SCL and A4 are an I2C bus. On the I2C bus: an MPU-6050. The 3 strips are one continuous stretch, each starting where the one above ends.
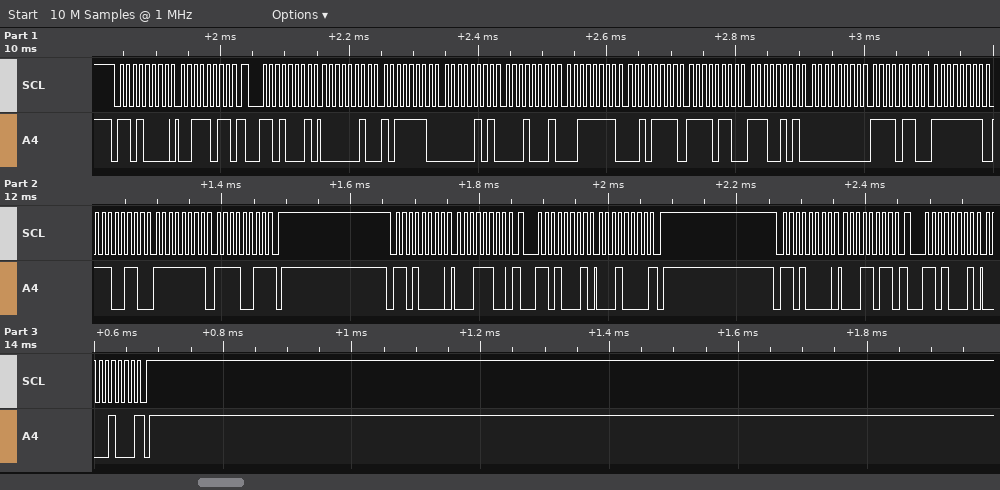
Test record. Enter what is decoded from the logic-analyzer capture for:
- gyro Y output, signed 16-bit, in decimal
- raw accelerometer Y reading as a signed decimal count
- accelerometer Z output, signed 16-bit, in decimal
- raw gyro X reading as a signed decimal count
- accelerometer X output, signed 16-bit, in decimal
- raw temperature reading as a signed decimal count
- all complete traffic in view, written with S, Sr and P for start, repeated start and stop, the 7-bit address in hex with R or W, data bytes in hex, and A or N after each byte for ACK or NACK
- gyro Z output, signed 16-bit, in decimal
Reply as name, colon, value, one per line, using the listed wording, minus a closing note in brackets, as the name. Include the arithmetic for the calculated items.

gyro Y output, signed 16-bit, in decimal: 0xFFE6 = -26
raw accelerometer Y reading as a signed decimal count: 0x0511 = 1297
accelerometer Z output, signed 16-bit, in decimal: 0x3F2F = 16175
raw gyro X reading as a signed decimal count: 0x00F6 = 246
accelerometer X output, signed 16-bit, in decimal: 0x02BE = 702
raw temperature reading as a signed decimal count: 0xF6E5 = -2331
all complete traffic in view, written with S, Sr and P for start, repeated start and stop, the 7-bit address in hex with R or W, data bytes in hex, and A or N after each byte for ACK or NACK: S 68W A 3B A Sr 68R A 02 A BE A 05 A 11 A 3F A 2F A F6 A E5 A 00 A F6 A FF A E6 A FF A F3 N P S 68W A 1C A Sr 68R A 10 N P S 68W A 1B A Sr 68R A 08 N P
gyro Z output, signed 16-bit, in decimal: 0xFFF3 = -13
